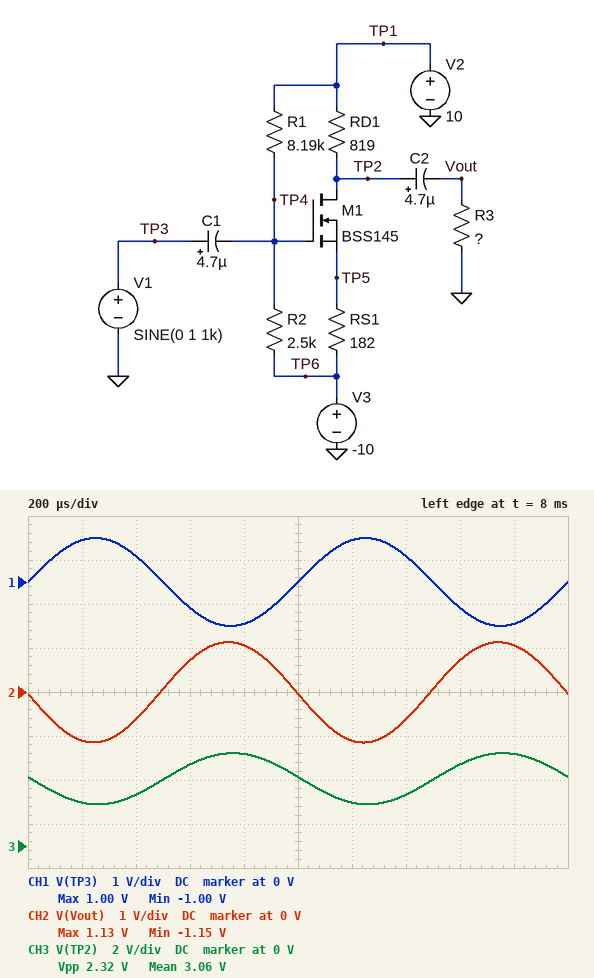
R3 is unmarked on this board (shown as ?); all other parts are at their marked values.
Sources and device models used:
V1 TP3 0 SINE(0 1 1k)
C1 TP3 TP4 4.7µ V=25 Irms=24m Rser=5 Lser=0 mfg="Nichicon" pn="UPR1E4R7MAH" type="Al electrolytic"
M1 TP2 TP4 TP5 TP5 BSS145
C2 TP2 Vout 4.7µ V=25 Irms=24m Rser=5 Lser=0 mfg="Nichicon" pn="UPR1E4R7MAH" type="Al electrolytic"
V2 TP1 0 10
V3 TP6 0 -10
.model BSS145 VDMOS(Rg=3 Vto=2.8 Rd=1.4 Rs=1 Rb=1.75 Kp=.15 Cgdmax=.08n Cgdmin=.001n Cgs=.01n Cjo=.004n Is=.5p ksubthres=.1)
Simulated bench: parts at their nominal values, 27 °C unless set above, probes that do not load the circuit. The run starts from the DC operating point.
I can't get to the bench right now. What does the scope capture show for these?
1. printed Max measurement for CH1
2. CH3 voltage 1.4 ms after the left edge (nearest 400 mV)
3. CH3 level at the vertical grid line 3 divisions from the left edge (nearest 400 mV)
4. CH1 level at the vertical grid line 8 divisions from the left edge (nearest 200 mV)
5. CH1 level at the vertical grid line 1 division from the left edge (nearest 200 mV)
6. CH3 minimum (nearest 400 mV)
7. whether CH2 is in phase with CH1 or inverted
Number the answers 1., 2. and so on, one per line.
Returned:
1. 1.00 V
2. 2.4 V
3. 3.6 V
4. -600 mV
5. 1.0 V
6. 2.0 V
7. inverted
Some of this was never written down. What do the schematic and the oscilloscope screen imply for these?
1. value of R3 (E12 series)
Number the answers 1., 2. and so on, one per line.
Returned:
1. 330 Ω
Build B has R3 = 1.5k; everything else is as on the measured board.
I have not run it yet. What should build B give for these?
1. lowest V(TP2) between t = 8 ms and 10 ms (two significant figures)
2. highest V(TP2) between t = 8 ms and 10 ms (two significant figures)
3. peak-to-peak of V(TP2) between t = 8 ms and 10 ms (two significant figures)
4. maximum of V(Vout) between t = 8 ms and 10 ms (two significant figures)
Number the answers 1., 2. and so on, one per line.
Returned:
1. 460 mV
2. 5.6 V
3. 5.2 V
4. 2.6 V
